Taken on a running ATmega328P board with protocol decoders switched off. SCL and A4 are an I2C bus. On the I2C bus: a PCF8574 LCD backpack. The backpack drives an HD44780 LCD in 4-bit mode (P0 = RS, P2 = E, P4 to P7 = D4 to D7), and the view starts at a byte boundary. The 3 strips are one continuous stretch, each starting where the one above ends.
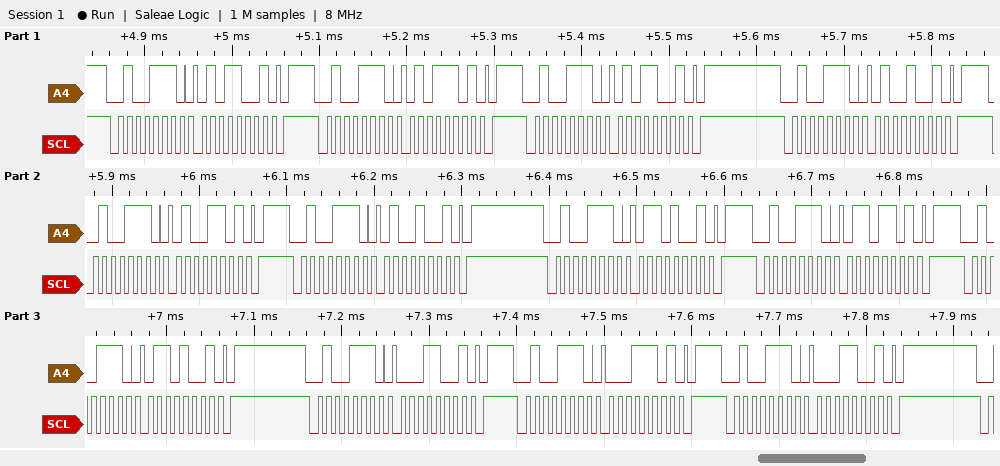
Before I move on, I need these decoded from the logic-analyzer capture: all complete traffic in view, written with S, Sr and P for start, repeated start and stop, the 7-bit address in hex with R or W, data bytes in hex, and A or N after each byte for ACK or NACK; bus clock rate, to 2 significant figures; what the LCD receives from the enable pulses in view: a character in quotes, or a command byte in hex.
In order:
S 27W A 59 A P S 27W A 5D A P S 27W A 59 A P S 27W A 49 A P S 27W A 4D A P S 27W A 49 A P S 27W A 69 A P S 27W A 6D A P S 27W A 69 A P S 27W A 19 A P S 27W A 1D A P S 27W A 19 A P
100 kHz
'T' 'a'
